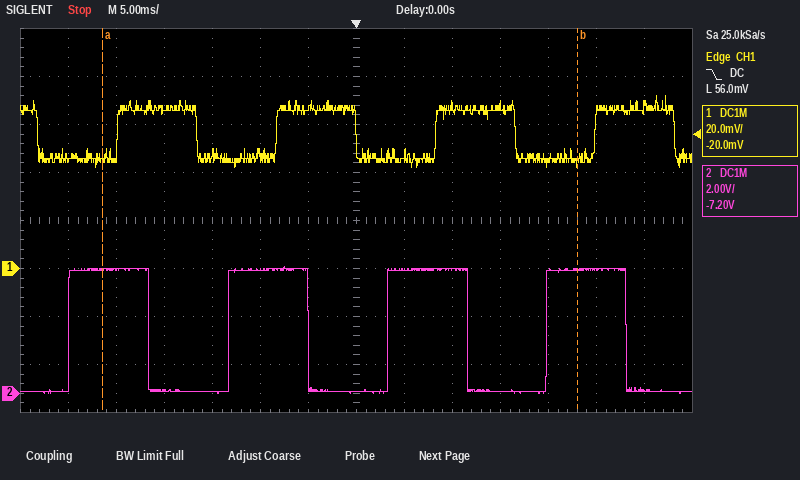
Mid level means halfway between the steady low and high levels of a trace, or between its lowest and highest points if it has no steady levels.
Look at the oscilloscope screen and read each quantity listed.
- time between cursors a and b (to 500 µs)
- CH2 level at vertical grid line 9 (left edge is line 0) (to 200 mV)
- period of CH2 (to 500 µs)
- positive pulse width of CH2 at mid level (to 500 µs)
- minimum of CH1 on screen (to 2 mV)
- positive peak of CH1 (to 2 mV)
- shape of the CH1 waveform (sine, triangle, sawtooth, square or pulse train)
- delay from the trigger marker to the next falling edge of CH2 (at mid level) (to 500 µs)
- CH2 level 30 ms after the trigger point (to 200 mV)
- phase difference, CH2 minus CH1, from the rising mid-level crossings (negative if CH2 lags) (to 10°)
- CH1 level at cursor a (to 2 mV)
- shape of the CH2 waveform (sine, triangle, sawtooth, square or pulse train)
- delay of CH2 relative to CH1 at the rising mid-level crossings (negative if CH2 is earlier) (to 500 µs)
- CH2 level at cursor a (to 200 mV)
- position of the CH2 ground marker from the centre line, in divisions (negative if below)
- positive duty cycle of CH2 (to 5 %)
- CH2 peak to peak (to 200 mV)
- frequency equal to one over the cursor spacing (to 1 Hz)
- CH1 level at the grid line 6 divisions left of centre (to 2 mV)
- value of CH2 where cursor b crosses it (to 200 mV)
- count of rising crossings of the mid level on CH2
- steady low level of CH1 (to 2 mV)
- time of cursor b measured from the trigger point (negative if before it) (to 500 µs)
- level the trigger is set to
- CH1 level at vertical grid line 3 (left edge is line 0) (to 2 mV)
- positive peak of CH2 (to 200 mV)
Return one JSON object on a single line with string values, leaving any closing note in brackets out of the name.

{"time between cursors a and b": "49.5 ms", "CH2 level at vertical grid line 9 (left edge is line 0)": "5.2 V", "period of CH2": "16.5 ms", "positive pulse width of CH2 at mid level": "8.5 ms", "minimum of CH1 on screen": "42 mV", "positive peak of CH1": "72 mV", "shape of the CH1 waveform": "square", "delay from the trigger marker to the next falling edge of CH2 (at mid level)": "11.5 ms", "CH2 level 30 ms after the trigger point": "200 mV", "phase difference, CH2 minus CH1, from the rising mid-level crossings (negative if CH2 lags)": "+110°", "CH1 level at cursor a": "46 mV", "shape of the CH2 waveform": "square", "delay of CH2 relative to CH1 at the rising mid-level crossings (negative if CH2 is earlier)": "-5.0 ms", "CH2 level at cursor a": "5.2 V", "position of the CH2 ground marker from the centre line, in divisions": "-3.6 div", "positive duty cycle of CH2": "50 %", "CH2 peak to peak": "5.2 V", "frequency equal to one over the cursor spacing": "20 Hz", "CH1 level at the grid line 6 divisions left of centre": "46 mV", "value of CH2 where cursor b crosses it": "5.2 V", "count of rising crossings of the mid level on CH2": "4", "steady low level of CH1": "46 mV", "time of cursor b measured from the trigger point (negative if before it)": "+23.0 ms", "level the trigger is set to": "56.0 mV", "CH1 level at vertical grid line 3 (left edge is line 0)": "66 mV", "positive peak of CH2": "5.2 V"}
